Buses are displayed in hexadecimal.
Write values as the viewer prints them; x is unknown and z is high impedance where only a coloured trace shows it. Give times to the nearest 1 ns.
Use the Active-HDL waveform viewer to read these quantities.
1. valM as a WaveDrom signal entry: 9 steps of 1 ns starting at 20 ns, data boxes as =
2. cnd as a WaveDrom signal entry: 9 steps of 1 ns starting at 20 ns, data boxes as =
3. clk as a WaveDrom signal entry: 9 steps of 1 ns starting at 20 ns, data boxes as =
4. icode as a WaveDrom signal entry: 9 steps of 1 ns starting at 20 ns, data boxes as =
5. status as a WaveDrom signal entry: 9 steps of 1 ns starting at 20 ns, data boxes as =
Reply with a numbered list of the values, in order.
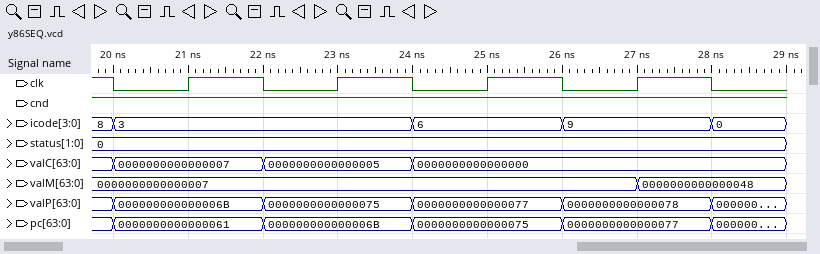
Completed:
1. {name: 'valM', wave: '=......=.', data: '0000000000000007 0000000000000048'}
2. {name: 'cnd', wave: '1........'}
3. {name: 'clk', wave: '010101010'}
4. {name: 'icode', wave: '=...=.=.=', data: '3 6 9 0'}
5. {name: 'status', wave: '=........', data: '0'}
